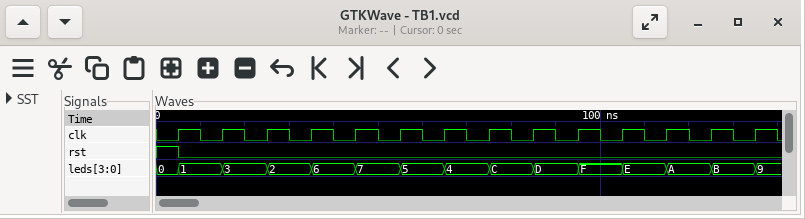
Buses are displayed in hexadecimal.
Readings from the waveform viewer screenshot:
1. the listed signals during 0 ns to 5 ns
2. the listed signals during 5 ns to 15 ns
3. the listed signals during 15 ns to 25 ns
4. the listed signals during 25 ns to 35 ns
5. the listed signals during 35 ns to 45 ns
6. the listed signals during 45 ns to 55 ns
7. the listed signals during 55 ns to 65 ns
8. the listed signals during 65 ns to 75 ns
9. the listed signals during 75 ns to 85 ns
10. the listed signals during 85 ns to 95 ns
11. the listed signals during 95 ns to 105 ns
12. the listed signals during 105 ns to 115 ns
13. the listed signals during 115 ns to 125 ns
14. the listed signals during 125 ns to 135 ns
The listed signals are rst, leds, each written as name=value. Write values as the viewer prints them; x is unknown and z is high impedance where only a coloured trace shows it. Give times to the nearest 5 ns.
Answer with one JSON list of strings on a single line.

["rst=1, leds=0", "rst=0, leds=1", "rst=0, leds=3", "rst=0, leds=2", "rst=0, leds=6", "rst=0, leds=7", "rst=0, leds=5", "rst=0, leds=4", "rst=0, leds=C", "rst=0, leds=D", "rst=0, leds=F", "rst=0, leds=E", "rst=0, leds=A", "rst=0, leds=B"]
